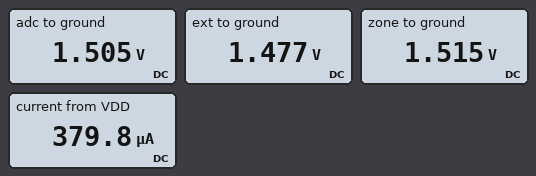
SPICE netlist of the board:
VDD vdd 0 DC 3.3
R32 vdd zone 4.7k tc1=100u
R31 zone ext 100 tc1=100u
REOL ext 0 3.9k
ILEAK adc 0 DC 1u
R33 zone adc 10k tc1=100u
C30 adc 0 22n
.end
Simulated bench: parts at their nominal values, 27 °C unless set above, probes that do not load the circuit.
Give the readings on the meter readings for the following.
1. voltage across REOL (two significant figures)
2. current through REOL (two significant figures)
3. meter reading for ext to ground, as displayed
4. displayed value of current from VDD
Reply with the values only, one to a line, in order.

1.5 V
380 µA
1.477 V
379.8 µA
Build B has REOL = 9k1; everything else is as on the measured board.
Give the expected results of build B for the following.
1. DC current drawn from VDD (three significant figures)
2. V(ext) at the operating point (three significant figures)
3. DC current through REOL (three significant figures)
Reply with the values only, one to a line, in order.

238 µA
2.16 V
237 µA
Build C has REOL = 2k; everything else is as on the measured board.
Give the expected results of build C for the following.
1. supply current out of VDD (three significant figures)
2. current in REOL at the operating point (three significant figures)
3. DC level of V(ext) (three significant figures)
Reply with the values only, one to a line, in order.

486 µA
485 µA
969 mV
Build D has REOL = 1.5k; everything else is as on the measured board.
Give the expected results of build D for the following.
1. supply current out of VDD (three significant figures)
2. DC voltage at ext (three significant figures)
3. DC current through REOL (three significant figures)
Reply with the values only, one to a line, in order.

524 µA
785 mV
523 µA
